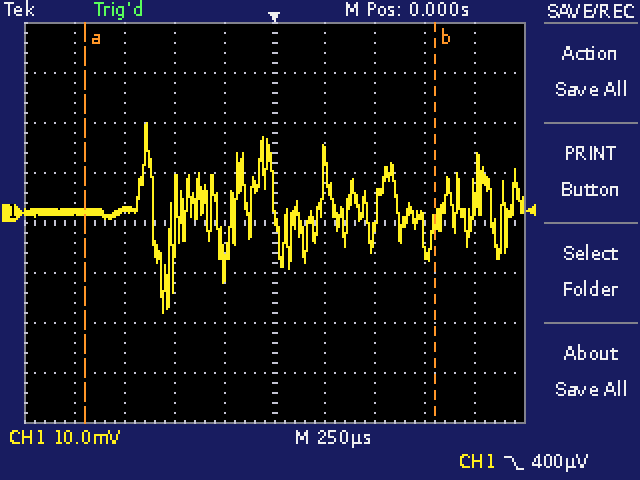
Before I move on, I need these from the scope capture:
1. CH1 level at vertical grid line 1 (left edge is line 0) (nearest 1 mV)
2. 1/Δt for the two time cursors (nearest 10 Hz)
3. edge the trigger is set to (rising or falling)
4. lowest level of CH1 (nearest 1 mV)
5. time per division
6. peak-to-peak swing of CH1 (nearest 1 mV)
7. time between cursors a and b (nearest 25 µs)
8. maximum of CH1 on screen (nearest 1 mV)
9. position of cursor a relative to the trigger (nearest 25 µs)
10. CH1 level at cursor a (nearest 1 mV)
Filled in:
0 mV
570 Hz
falling
-20 mV
250 µs
38 mV
1.750 ms
18 mV
-950 µs
0 mV
